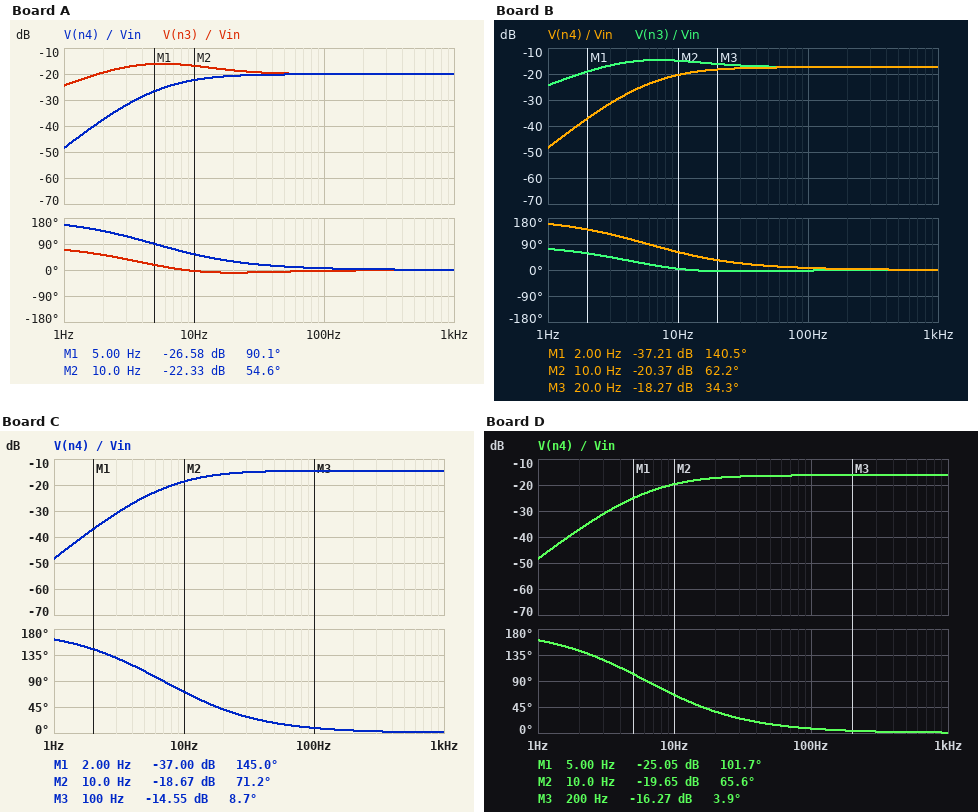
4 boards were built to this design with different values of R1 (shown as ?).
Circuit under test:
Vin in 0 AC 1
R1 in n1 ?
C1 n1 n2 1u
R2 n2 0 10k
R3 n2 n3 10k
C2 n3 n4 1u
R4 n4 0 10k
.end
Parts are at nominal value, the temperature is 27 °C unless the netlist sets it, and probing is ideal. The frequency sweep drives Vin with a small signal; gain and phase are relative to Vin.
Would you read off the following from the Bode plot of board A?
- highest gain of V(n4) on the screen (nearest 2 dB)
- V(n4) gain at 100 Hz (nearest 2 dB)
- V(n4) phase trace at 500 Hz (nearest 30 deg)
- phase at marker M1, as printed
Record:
-20 dB
-20 dB
0 deg
90.1 deg
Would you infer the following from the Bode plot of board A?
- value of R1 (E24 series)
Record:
27 kΩ
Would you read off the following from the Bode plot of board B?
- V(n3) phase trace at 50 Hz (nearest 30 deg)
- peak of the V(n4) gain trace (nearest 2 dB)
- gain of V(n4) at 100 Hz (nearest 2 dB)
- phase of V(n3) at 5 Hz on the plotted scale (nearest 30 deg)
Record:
0 deg
-18 dB
-18 dB
30 deg
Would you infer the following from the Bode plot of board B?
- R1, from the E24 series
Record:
18 kΩ
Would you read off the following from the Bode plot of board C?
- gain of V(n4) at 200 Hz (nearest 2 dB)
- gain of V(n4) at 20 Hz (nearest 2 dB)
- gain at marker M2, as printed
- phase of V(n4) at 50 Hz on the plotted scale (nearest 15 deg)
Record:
-14 dB
-16 dB
-18.67 dB
15 deg
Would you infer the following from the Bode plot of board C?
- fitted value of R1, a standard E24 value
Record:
11 kΩ
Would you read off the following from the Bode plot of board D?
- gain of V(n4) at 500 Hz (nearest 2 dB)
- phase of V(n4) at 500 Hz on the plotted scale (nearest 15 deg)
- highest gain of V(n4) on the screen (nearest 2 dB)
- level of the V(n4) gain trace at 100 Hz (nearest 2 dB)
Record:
-16 dB
0 deg
-16 dB
-16 dB
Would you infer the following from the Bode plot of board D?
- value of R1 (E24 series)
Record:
15 kΩ
